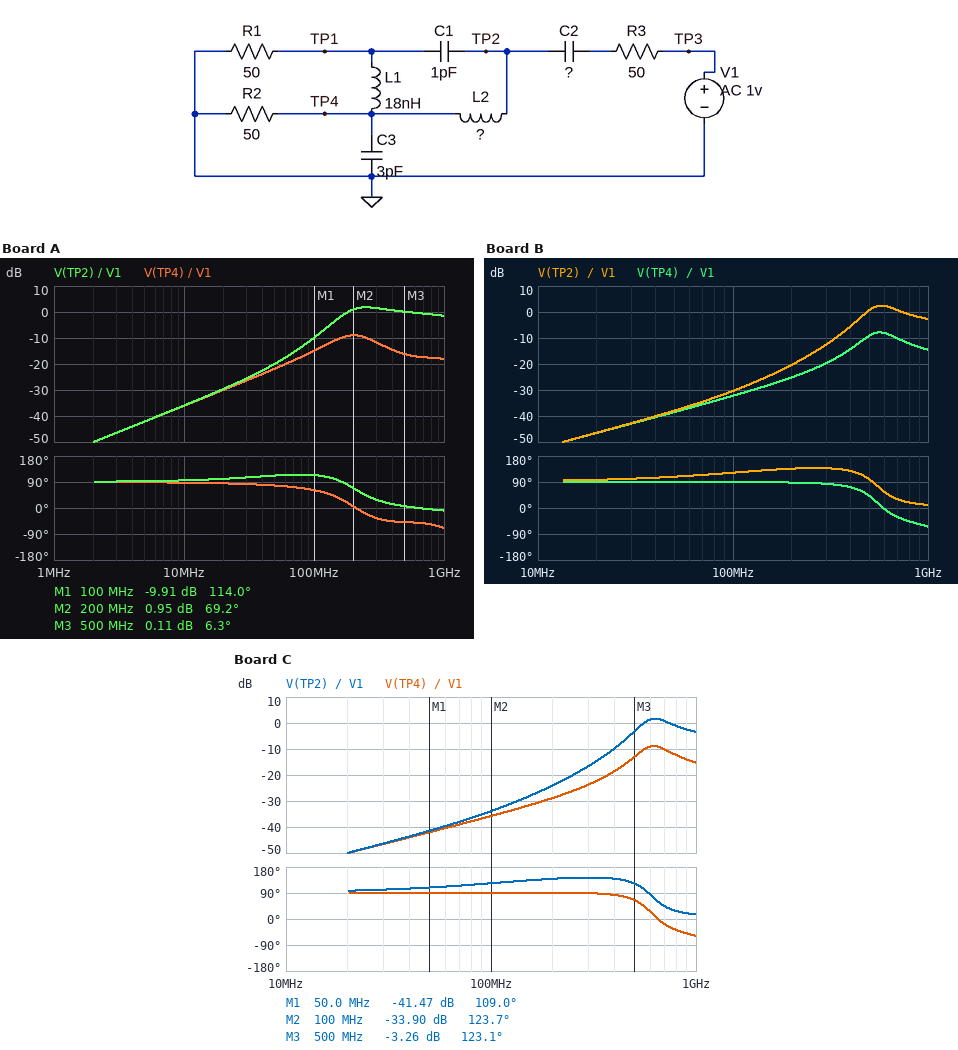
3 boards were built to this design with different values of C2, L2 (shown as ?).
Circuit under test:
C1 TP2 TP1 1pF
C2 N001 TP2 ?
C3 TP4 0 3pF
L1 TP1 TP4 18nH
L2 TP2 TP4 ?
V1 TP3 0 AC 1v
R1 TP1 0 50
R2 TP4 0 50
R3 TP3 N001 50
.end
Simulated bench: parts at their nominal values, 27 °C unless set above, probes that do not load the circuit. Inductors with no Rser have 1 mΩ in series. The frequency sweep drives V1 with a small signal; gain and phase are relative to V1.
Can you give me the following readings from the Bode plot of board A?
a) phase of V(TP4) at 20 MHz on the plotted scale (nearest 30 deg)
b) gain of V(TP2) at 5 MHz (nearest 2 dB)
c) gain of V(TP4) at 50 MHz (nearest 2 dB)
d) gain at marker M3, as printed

90 deg
-42 dB
-22 dB
0.11 dB
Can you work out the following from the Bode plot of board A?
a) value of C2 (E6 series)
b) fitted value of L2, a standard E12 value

10 pF
56 nH
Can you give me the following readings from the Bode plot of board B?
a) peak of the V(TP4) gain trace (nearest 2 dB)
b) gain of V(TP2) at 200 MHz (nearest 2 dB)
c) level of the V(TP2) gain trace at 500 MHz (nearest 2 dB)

-8 dB
-20 dB
0 dB
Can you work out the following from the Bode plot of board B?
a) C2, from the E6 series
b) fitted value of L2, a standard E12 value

1.5 pF
27 nH
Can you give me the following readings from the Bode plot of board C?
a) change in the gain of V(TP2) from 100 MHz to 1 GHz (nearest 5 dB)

30 dB
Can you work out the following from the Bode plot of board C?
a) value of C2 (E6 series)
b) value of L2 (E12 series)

1 pF
27 nH
